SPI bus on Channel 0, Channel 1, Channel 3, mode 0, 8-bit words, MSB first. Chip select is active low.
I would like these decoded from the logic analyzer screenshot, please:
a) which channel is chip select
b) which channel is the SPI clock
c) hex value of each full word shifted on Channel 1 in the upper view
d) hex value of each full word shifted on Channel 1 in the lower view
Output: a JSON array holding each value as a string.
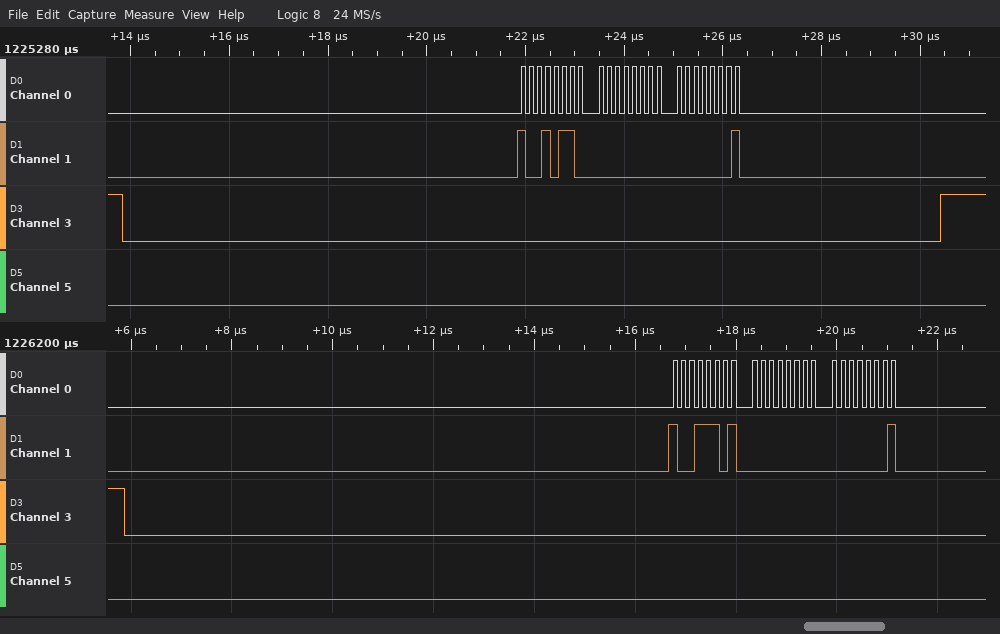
["Channel 3", "Channel 0", "96, 00, 01", "9D, 00, 01"]
